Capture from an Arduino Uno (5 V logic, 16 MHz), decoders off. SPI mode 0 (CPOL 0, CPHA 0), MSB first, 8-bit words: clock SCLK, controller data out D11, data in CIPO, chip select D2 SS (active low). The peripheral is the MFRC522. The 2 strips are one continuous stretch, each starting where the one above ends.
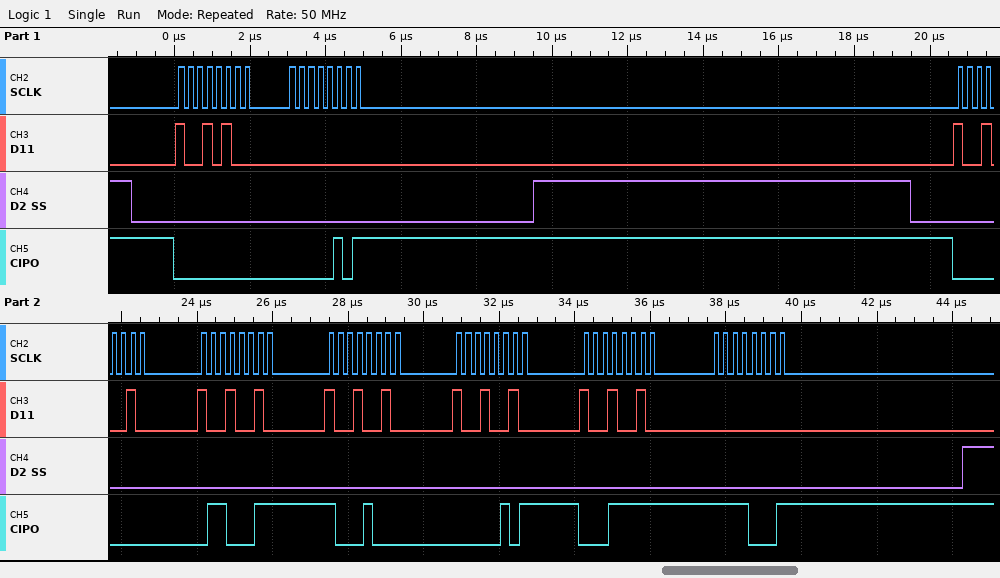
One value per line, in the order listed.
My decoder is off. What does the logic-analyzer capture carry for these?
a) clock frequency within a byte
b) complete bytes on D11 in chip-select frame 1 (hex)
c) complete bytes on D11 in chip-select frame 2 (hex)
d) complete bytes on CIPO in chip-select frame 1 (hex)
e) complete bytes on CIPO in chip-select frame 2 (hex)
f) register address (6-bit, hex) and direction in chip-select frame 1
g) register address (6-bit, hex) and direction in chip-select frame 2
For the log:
4 MHz
0x94 0x00
0x92 0x92 0x92 0x92 0x92 0x00
0x00 0x05
0x00 0x63 0x88 0x05 0x1F 0xF1
0x0A read
0x09 read
